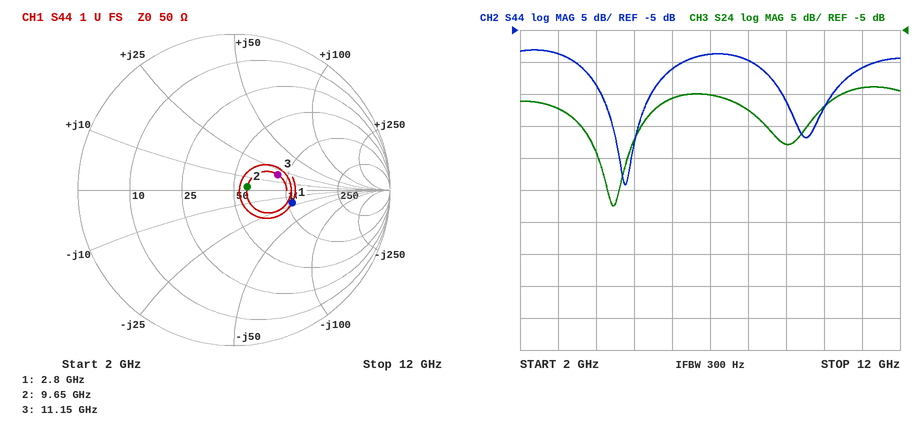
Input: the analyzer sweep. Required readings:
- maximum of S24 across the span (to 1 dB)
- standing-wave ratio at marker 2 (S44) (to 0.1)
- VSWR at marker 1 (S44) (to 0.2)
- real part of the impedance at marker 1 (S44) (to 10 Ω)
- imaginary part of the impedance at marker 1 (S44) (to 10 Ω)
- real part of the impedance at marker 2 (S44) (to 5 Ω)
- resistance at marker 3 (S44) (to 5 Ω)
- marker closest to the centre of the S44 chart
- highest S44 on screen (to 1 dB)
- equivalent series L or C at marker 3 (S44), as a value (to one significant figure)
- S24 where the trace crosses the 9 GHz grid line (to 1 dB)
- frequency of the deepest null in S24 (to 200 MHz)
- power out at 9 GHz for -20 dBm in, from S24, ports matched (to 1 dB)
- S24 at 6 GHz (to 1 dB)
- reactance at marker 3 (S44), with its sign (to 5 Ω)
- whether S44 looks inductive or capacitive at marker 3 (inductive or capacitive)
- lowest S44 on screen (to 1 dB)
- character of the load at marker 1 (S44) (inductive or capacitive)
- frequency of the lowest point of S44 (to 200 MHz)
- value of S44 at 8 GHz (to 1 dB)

-14 dB
1.2
2.2
110 Ω
-20 Ω
60 Ω
85 Ω
marker 2
-8 dB
300 pH
-23 dB
4.4 GHz
-43 dBm
-16 dB
+20 Ω
inductive
-29 dB
capacitive
4.8 GHz
-10 dB
